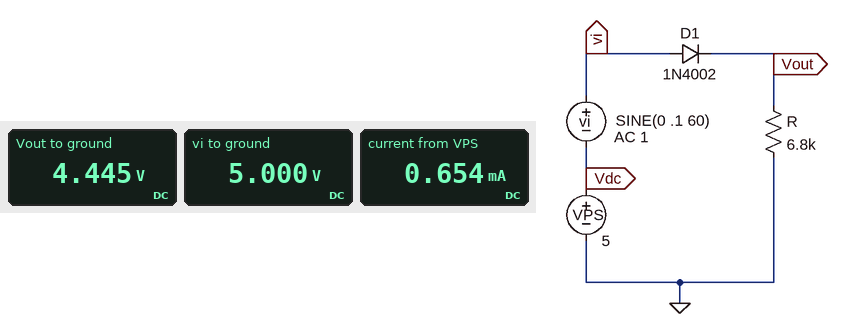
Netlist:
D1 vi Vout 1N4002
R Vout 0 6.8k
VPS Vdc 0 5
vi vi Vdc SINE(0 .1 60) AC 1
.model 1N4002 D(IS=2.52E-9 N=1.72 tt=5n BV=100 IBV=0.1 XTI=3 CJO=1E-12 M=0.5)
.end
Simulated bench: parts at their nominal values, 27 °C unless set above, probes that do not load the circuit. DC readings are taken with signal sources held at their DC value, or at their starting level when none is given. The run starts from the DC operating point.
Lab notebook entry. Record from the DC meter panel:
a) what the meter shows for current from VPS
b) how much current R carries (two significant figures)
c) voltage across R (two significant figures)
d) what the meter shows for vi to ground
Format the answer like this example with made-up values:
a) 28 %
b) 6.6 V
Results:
a) 0.654 mA
b) 650 µA
c) 4.4 V
d) 5.000 V
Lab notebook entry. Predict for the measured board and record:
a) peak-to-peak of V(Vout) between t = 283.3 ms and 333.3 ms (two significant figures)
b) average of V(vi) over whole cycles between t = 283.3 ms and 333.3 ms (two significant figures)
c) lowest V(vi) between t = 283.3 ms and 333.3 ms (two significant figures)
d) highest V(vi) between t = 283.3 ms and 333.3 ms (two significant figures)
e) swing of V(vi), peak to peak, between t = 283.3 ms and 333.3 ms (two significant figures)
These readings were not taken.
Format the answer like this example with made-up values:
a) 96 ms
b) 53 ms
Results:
a) 200 mV
b) 5.0 V
c) 4.9 V
d) 5.1 V
e) 200 mV
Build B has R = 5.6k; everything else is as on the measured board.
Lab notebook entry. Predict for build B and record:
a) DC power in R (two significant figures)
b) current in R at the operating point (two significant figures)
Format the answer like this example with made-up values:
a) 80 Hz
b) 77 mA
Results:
a) 3.5 mW
b) 790 µA
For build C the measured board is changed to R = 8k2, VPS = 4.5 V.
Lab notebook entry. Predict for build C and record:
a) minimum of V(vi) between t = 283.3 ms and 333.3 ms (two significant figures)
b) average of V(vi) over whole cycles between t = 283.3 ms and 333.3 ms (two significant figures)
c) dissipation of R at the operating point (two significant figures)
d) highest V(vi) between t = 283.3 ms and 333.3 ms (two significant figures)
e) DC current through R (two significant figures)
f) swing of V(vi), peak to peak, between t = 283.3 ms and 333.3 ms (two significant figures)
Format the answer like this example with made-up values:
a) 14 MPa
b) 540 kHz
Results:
a) 4.4 V
b) 4.5 V
c) 1.9 mW
d) 4.6 V
e) 480 µA
f) 200 mV
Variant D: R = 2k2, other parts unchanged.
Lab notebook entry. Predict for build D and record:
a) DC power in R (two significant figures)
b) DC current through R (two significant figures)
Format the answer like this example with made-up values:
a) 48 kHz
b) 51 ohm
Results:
a) 8.8 mW
b) 2.0 mA
